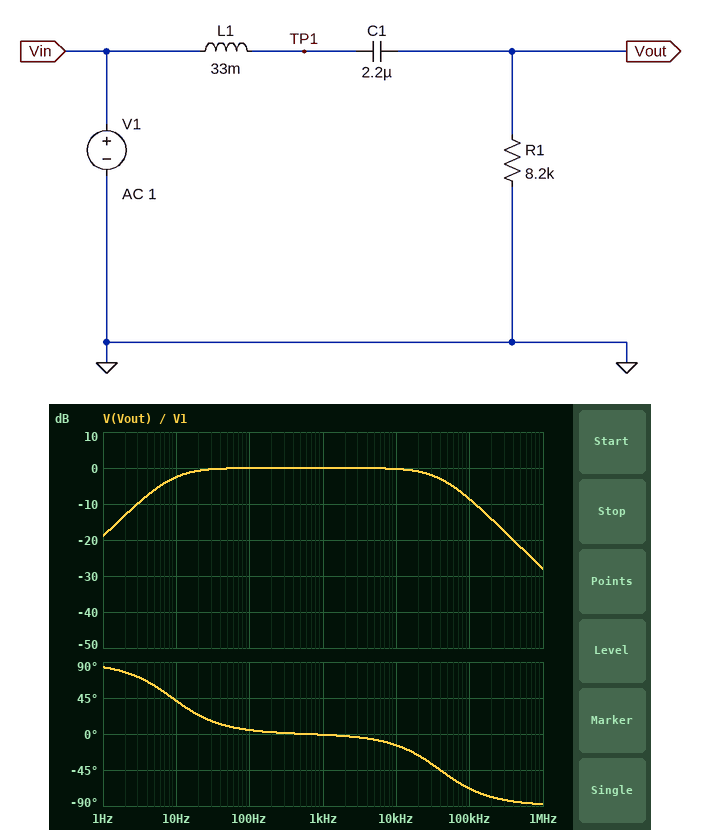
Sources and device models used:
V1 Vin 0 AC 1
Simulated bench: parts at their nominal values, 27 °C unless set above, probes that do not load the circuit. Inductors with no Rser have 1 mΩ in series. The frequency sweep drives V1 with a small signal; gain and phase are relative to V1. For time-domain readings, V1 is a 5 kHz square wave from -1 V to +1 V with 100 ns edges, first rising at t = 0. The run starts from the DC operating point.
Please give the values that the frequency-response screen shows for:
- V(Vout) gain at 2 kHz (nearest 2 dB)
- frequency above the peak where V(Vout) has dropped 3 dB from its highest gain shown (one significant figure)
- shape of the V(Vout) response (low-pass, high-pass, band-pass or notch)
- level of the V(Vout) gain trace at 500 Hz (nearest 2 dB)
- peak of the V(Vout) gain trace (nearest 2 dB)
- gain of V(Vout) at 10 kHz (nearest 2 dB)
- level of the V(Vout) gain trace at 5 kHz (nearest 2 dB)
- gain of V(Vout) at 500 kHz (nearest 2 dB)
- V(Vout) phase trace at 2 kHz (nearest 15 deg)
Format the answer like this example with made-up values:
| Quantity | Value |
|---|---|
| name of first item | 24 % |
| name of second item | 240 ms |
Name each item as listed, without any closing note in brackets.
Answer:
| Quantity | Value |
|---|---|
| V(Vout) gain at 2 kHz | 0 dB |
| frequency above the peak where V(Vout) has dropped 3 dB from its highest gain shown | 40 kHz |
| shape of the V(Vout) response | band-pass |
| level of the V(Vout) gain trace at 500 Hz | 0 dB |
| peak of the V(Vout) gain trace | 0 dB |
| gain of V(Vout) at 10 kHz | 0 dB |
| level of the V(Vout) gain trace at 5 kHz | 0 dB |
| gain of V(Vout) at 500 kHz | -22 dB |
| V(Vout) phase trace at 2 kHz | 0 deg |
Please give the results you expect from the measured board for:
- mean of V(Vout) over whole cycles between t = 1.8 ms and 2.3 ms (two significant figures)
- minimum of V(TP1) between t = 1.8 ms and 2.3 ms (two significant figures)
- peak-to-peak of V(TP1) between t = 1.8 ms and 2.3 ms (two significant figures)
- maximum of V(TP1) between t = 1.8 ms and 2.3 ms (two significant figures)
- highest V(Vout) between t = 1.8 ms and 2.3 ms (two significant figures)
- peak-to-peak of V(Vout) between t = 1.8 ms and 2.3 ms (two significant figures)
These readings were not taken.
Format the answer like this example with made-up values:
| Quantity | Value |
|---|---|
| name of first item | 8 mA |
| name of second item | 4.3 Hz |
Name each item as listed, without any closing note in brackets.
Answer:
| Quantity | Value |
|---|---|
| mean of V(Vout) over whole cycles between t = 1.8 ms and 2.3 ms | 890 mV |
| minimum of V(TP1) between t = 1.8 ms and 2.3 ms | -1.0 V |
| peak-to-peak of V(TP1) between t = 1.8 ms and 2.3 ms | 2.0 V |
| maximum of V(TP1) between t = 1.8 ms and 2.3 ms | 1.0 V |
| highest V(Vout) between t = 1.8 ms and 2.3 ms | 1.9 V |
| peak-to-peak of V(Vout) between t = 1.8 ms and 2.3 ms | 2.0 V |
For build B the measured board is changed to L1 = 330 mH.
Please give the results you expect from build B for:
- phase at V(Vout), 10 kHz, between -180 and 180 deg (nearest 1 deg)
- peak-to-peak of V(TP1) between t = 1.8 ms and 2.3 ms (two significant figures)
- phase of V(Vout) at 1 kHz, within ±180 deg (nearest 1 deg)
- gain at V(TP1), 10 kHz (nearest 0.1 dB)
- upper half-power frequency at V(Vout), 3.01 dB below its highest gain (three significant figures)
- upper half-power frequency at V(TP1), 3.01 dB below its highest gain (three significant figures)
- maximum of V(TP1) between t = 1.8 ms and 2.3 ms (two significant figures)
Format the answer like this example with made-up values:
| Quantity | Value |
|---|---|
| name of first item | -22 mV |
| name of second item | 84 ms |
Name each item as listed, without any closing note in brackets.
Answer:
| Quantity | Value |
|---|---|
| phase at V(Vout), 10 kHz, between -180 and 180 deg | -68 deg |
| peak-to-peak of V(TP1) between t = 1.8 ms and 2.3 ms | 1.7 V |
| phase of V(Vout) at 1 kHz, within ±180 deg | -14 deg |
| gain at V(TP1), 10 kHz | -8.7 dB |
| upper half-power frequency at V(Vout), 3.01 dB below its highest gain | 3.96 kHz |
| upper half-power frequency at V(TP1), 3.01 dB below its highest gain | 3.95 kHz |
| maximum of V(TP1) between t = 1.8 ms and 2.3 ms | 850 mV |
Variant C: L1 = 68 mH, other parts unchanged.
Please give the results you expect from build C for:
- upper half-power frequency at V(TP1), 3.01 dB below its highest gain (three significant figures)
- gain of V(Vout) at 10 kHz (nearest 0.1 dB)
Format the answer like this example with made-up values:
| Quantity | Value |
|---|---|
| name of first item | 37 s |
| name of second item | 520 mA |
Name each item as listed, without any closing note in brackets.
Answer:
| Quantity | Value |
|---|---|
| upper half-power frequency at V(TP1), 3.01 dB below its highest gain | 19.2 kHz |
| gain of V(Vout) at 10 kHz | -1.0 dB |
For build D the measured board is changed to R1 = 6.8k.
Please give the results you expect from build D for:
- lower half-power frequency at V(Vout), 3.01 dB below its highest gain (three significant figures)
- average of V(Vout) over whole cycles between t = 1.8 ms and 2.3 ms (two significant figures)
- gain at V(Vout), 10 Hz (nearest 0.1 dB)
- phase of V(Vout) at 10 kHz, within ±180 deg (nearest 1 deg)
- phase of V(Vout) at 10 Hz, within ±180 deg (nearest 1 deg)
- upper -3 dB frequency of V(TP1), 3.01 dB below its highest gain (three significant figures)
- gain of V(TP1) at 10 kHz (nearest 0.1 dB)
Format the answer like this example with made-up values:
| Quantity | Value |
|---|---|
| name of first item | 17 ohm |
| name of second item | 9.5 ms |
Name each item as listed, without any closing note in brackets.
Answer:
| Quantity | Value |
|---|---|
| lower half-power frequency at V(Vout), 3.01 dB below its highest gain | 10.6 Hz |
| average of V(Vout) over whole cycles between t = 1.8 ms and 2.3 ms | 870 mV |
| gain at V(Vout), 10 Hz | -3.3 dB |
| phase of V(Vout) at 10 kHz, within ±180 deg | -17 deg |
| phase of V(Vout) at 10 Hz, within ±180 deg | 47 deg |
| upper -3 dB frequency of V(TP1), 3.01 dB below its highest gain | 32.8 kHz |
| gain of V(TP1) at 10 kHz | -0.4 dB |
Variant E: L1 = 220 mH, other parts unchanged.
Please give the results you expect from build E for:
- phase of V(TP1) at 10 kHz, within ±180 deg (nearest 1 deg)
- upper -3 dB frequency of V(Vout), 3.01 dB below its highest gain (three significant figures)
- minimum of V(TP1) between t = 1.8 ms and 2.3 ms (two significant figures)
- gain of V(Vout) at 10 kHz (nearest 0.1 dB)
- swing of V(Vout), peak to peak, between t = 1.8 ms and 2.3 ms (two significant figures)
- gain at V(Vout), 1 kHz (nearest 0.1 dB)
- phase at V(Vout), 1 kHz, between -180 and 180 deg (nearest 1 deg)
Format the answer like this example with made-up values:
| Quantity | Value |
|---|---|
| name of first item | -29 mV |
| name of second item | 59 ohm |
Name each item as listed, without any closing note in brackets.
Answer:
| Quantity | Value |
|---|---|
| phase of V(TP1) at 10 kHz, within ±180 deg | -59 deg |
| upper -3 dB frequency of V(Vout), 3.01 dB below its highest gain | 5.94 kHz |
| minimum of V(TP1) between t = 1.8 ms and 2.3 ms | -950 mV |
| gain of V(Vout) at 10 kHz | -5.8 dB |
| swing of V(Vout), peak to peak, between t = 1.8 ms and 2.3 ms | 1.9 V |
| gain at V(Vout), 1 kHz | -0.1 dB |
| phase at V(Vout), 1 kHz, between -180 and 180 deg | -9 deg |
